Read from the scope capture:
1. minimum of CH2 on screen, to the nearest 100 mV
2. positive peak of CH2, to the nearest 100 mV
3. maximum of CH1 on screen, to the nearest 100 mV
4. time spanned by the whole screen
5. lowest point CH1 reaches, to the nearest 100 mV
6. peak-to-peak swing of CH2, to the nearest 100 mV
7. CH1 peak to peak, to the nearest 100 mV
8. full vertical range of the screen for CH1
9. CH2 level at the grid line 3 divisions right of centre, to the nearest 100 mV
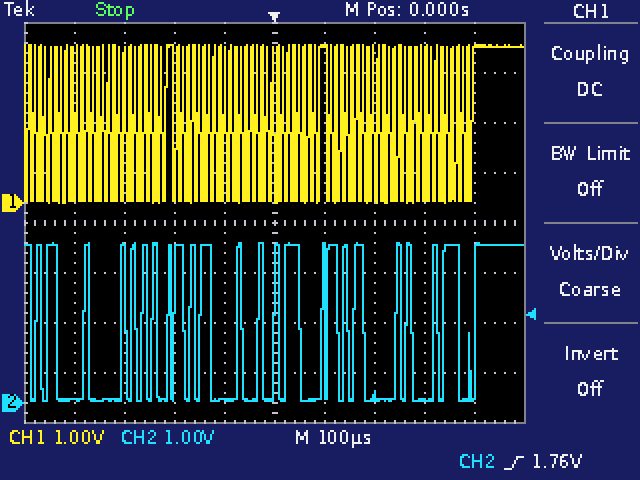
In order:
0.0 V
3.2 V
3.2 V
1 ms
0.0 V
3.2 V
3.2 V
8 V
100 mV
